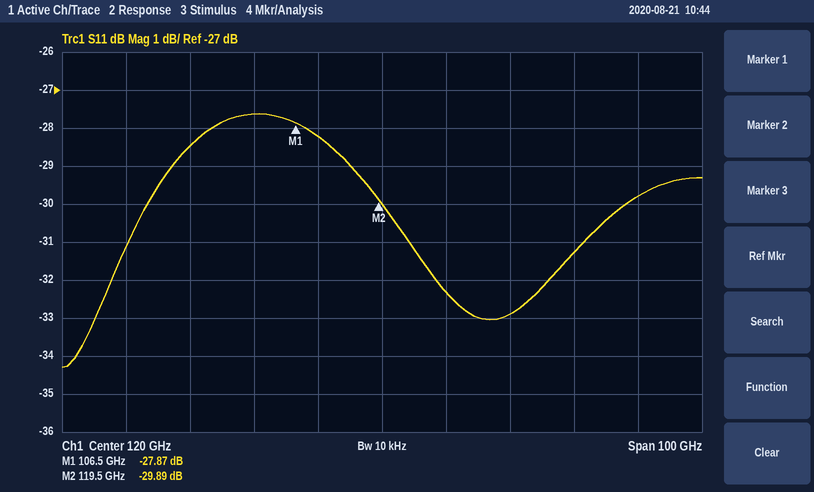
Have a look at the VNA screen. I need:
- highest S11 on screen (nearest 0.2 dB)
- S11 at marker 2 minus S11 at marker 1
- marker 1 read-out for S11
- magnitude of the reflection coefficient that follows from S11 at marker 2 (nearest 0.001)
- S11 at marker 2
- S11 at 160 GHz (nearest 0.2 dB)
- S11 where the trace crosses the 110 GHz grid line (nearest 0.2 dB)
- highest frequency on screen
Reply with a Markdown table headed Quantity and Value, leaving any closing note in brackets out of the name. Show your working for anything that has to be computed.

| Quantity | Value |
|---|---|
| highest S11 on screen | -27.6 dB |
| S11 at marker 2 minus S11 at marker 1 | -29.89 − (-27.87) = -2.02 dB |
| marker 1 read-out for S11 | -27.87 dB |
| magnitude of the reflection coefficient that follows from S11 at marker 2 | 10^(-29.89/20) ≈ 0.032 |
| S11 at marker 2 | -29.89 dB |
| S11 at 160 GHz | -29.8 dB |
| S11 where the trace crosses the 110 GHz grid line | -28.2 dB |
| highest frequency on screen | 170 GHz |
